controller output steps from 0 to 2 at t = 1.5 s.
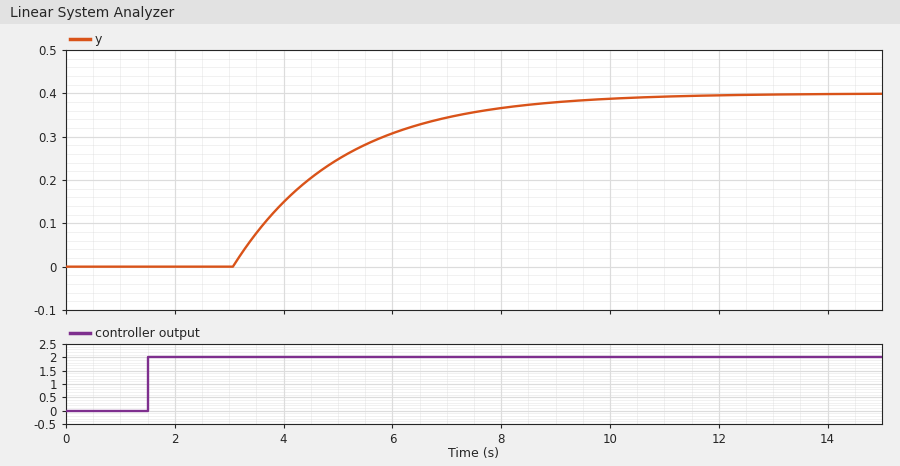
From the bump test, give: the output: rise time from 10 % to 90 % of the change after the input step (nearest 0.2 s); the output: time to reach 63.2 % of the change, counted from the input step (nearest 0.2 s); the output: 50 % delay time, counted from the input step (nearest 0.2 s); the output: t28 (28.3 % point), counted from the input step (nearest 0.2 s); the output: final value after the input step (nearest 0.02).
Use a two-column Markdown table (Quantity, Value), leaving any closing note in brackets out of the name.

| Quantity | Value |
|---|---|
| the output: rise time from 10 % to 90 % of the change after the input step | 4.4 s |
| the output: time to reach 63.2 % of the change, counted from the input step | 3.6 s |
| the output: 50 % delay time, counted from the input step | 3.0 s |
| the output: t28 (28.3 % point), counted from the input step | 2.2 s |
| the output: final value after the input step | 0.40 |
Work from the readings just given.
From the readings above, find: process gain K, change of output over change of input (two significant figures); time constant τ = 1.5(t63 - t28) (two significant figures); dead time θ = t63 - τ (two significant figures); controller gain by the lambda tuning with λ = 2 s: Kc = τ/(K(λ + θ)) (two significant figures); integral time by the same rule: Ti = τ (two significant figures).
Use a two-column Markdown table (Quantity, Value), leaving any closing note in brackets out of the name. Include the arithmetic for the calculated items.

| Quantity | Value |
|---|---|
| process gain K, change of output over change of input | (0.4 - 0) / 2 = 0.20 |
| time constant τ = 1.5(t63 - t28) | 1.5 × (3.6 - 2.2) = 2.1 s |
| dead time θ = t63 - τ | 3.6 - 2.1 = 1.5 s |
| controller gain by the lambda tuning with λ = 2 s: Kc = τ/(K(λ + θ)) | 2.1 / (0.2 × (2 + 1.5)) = 3.0 |
| integral time by the same rule: Ti = τ | 2.1 s |
